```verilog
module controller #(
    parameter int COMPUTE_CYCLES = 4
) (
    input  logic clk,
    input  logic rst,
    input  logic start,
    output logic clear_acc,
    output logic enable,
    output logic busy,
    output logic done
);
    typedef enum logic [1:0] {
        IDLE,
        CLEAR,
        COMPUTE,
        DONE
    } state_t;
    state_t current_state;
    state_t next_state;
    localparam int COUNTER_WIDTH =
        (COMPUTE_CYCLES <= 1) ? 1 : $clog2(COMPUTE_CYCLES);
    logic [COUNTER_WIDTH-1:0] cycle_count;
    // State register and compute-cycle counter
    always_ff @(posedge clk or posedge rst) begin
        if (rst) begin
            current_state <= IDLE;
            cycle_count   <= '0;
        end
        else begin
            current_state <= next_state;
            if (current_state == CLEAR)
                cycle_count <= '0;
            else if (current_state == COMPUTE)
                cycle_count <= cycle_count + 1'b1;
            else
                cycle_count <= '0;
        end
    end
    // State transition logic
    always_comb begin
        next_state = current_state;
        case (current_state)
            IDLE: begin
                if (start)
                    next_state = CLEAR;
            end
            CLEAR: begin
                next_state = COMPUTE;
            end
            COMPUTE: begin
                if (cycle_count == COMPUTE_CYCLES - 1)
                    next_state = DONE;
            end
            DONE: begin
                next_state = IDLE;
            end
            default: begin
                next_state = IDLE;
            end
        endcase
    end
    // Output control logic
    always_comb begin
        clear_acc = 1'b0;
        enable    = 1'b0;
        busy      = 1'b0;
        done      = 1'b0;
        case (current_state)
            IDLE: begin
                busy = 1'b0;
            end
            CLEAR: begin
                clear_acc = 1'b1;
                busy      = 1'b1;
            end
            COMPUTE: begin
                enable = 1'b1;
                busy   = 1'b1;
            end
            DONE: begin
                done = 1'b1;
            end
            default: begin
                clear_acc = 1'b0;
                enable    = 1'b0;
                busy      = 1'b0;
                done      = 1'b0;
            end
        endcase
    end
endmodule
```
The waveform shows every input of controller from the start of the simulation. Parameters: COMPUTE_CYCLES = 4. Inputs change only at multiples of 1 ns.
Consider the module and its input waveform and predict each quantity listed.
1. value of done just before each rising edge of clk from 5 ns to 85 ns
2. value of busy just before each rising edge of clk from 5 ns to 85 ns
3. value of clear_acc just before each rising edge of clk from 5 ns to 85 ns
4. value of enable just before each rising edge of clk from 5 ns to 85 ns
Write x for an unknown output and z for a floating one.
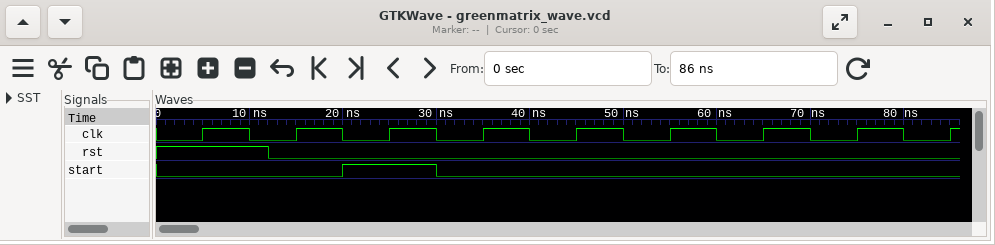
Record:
0 0 0 0 0 0 0 0 1
0 0 0 1 1 1 1 1 0
0 0 0 1 0 0 0 0 0
0 0 0 0 1 1 1 1 0
